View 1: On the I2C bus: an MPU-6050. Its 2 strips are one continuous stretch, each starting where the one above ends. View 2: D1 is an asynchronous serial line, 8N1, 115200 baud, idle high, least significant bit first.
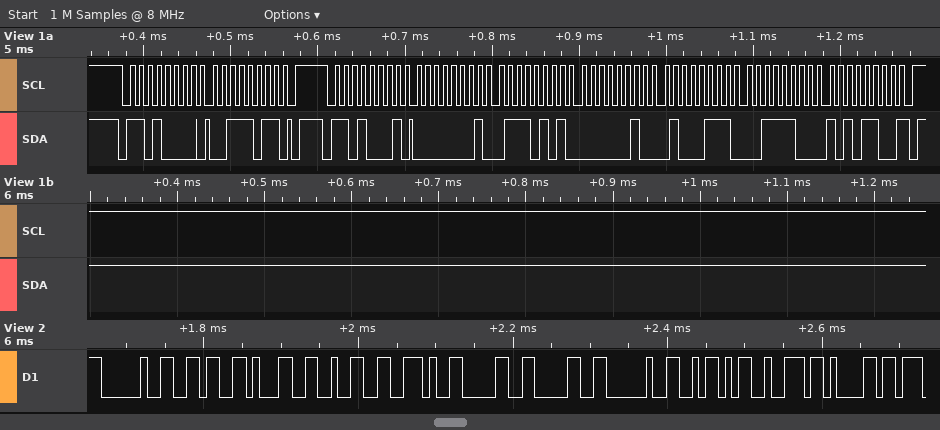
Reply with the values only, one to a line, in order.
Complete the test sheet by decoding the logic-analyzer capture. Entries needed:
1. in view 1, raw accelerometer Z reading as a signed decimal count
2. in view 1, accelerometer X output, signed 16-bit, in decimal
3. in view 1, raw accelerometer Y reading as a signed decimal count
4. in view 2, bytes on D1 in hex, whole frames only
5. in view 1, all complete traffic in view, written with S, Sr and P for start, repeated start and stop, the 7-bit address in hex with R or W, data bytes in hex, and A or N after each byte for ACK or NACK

15532
373
583
0x20 0x36 0x31 0x32 0x2E 0x30 0x30 0x20 0x5A 0x72 0x61
S 68W A 3B A P S 68R A 01 A 75 A 02 A 47 A 3C A AC N P
